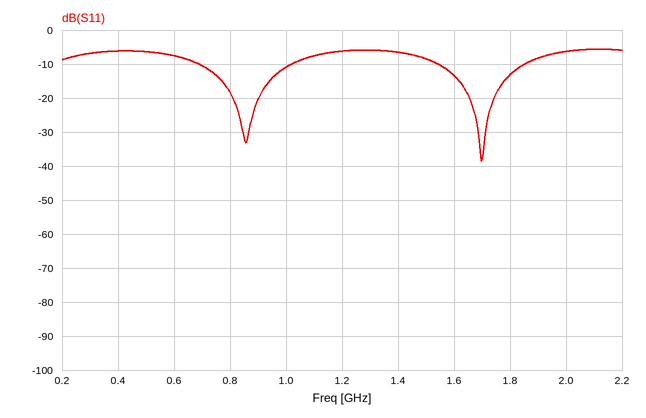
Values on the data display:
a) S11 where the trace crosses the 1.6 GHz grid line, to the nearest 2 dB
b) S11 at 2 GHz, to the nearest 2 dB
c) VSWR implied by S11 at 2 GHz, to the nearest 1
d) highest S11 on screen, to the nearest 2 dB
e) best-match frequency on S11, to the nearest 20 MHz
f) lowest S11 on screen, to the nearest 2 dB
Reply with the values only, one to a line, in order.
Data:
-14 dB
-6 dB
3
-6 dB
1.70 GHz
-38 dB
